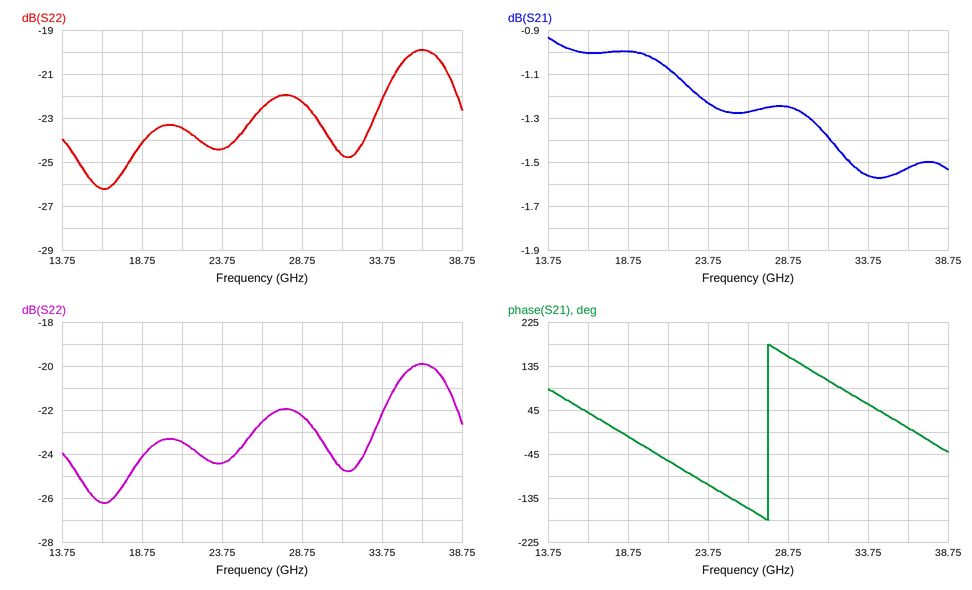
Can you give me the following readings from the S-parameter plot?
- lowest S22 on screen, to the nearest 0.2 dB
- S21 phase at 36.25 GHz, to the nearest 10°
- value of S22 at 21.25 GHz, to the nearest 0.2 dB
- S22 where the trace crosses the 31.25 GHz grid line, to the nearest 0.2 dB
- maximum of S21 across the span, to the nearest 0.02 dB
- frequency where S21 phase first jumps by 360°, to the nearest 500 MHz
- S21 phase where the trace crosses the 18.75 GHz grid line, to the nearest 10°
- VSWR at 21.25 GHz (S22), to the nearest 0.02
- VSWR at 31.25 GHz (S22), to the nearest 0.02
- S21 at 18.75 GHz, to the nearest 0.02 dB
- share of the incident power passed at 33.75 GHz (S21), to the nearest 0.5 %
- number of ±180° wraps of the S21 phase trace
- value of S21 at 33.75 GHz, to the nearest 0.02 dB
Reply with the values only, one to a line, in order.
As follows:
-26.2 dB
10°
-23.4 dB
-24.6 dB
-0.94 dB
27.5 GHz
-10°
1.14
1.12
-1.00 dB
70.0 %
1
-1.56 dB
